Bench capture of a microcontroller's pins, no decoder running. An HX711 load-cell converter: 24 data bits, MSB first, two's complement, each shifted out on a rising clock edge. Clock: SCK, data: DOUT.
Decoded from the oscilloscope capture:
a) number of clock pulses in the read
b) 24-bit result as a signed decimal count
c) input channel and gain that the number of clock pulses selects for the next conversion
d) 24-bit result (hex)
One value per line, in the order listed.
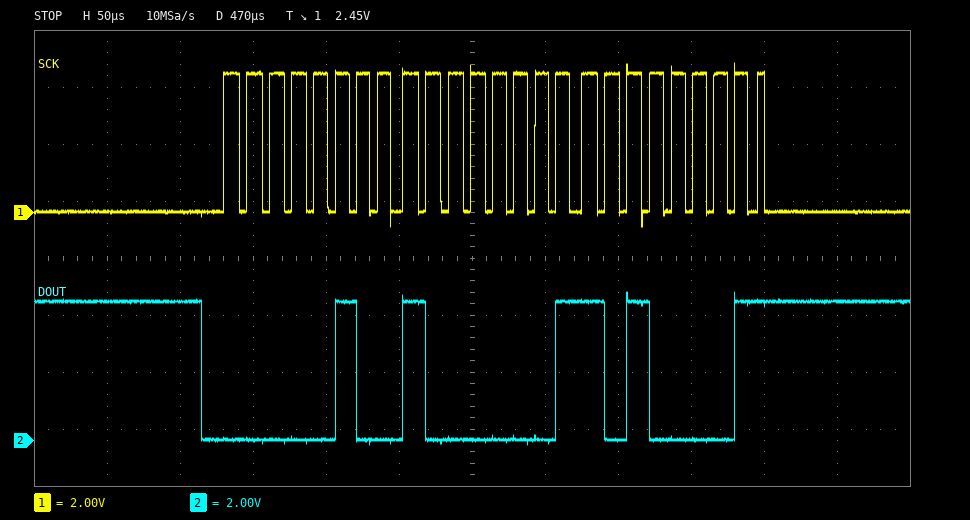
25
295329
channel A, gain 128
0x0481A1
